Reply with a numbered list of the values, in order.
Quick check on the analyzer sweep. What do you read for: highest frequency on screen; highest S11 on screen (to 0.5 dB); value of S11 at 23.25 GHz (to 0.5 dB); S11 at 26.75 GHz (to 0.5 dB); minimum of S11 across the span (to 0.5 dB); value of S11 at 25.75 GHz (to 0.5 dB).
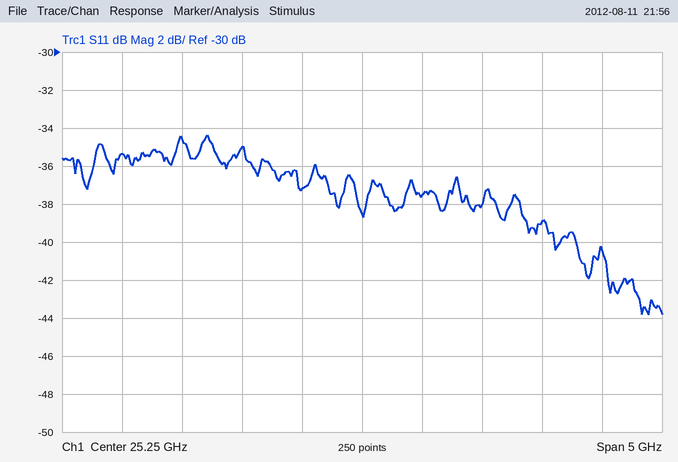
1. 27.75 GHz
2. -34.5 dB
3. -35.5 dB
4. -39.0 dB
5. -44.0 dB
6. -37.5 dB
